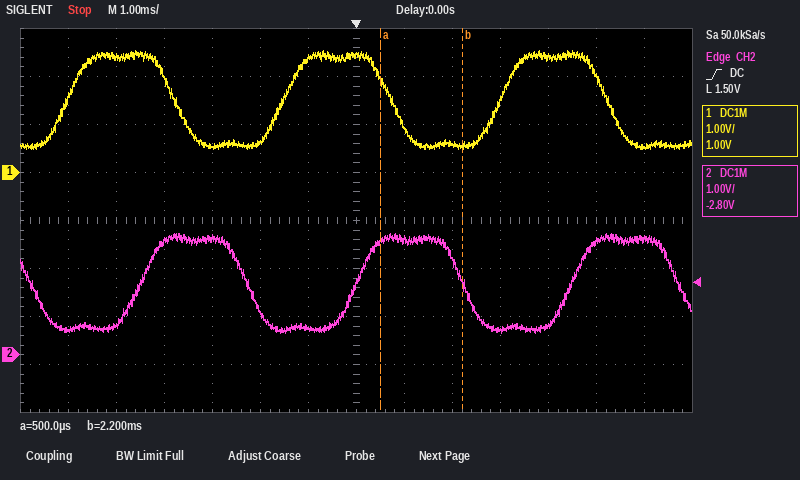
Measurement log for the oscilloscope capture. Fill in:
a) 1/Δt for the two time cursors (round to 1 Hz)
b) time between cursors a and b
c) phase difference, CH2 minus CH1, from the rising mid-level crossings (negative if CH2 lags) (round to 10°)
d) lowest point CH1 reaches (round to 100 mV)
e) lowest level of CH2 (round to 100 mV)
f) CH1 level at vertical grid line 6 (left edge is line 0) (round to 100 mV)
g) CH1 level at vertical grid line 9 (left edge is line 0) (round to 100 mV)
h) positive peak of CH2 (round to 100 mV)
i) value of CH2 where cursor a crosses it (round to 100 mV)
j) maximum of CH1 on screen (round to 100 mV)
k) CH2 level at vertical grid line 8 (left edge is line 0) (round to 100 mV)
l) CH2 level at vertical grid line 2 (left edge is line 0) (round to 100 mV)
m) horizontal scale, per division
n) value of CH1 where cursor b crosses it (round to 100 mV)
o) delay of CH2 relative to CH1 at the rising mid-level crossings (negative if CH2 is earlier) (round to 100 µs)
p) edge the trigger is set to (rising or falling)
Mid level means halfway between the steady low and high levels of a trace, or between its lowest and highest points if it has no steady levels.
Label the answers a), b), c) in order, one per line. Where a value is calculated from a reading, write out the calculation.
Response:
a) 1 / 1.7 ms ≈ 588 Hz
b) 2.2 ms − (500 µs) = 1.7 ms
c) -120°
d) 500 mV
e) 500 mV
f) 2.4 V
g) 600 mV
h) 2.5 V
i) 2.4 V
j) 2.5 V
k) 2.4 V
l) 600 mV
m) 1 ms
n) 600 mV
o) +1.5 ms
p) rising
